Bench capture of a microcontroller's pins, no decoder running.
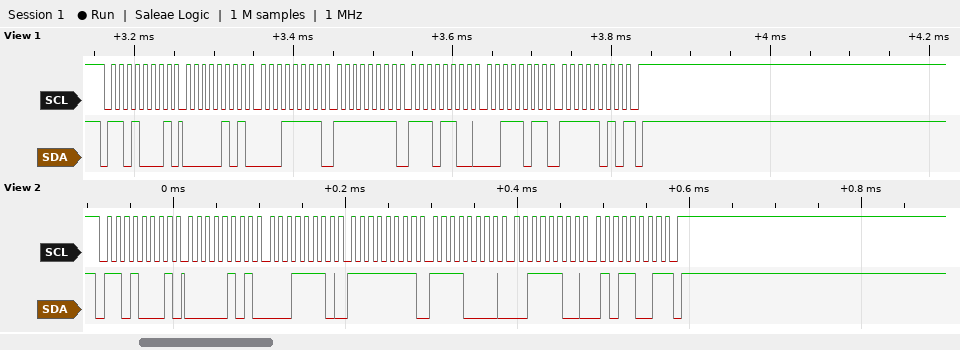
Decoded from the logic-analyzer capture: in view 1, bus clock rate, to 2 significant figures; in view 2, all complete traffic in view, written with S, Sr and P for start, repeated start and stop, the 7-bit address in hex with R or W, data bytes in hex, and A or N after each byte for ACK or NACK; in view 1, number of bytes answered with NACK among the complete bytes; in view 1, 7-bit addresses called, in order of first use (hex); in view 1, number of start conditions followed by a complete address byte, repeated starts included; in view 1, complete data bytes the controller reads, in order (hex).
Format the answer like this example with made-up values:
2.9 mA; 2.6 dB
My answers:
100 kHz; S 68R A 05 A 1E A FF A F0 A 3C A 59 N P; 1; 0x68; 1; 05 1F FF EC 3B FA
